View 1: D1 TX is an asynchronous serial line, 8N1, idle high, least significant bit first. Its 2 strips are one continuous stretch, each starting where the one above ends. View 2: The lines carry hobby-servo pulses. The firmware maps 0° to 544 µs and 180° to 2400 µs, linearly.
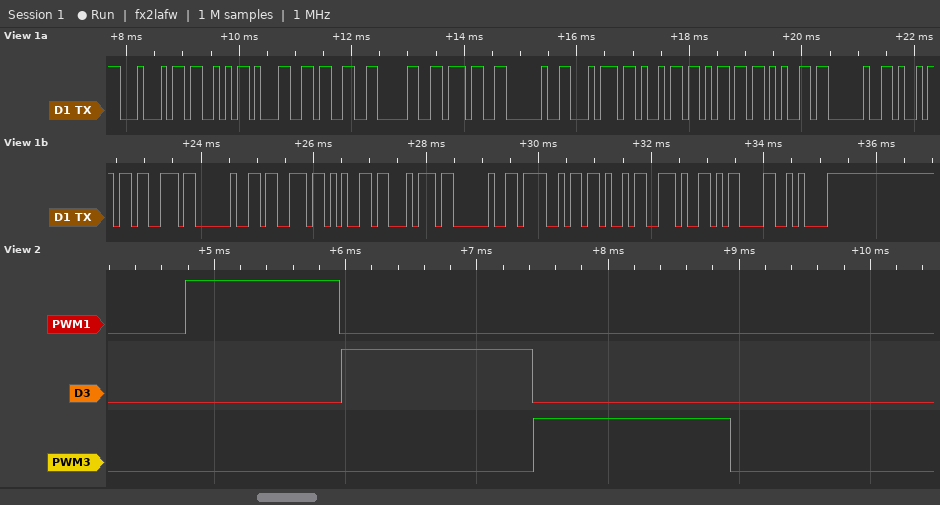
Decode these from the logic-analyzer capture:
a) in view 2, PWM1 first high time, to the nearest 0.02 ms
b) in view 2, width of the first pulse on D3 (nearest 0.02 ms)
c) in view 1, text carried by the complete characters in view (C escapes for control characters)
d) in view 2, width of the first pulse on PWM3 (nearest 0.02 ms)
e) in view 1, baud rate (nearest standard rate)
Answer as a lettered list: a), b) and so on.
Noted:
a) 1.18 ms
b) 1.46 ms
c) "DS1307 time is set OK.\r\n"
d) 1.50 ms
e) 9600 baud
